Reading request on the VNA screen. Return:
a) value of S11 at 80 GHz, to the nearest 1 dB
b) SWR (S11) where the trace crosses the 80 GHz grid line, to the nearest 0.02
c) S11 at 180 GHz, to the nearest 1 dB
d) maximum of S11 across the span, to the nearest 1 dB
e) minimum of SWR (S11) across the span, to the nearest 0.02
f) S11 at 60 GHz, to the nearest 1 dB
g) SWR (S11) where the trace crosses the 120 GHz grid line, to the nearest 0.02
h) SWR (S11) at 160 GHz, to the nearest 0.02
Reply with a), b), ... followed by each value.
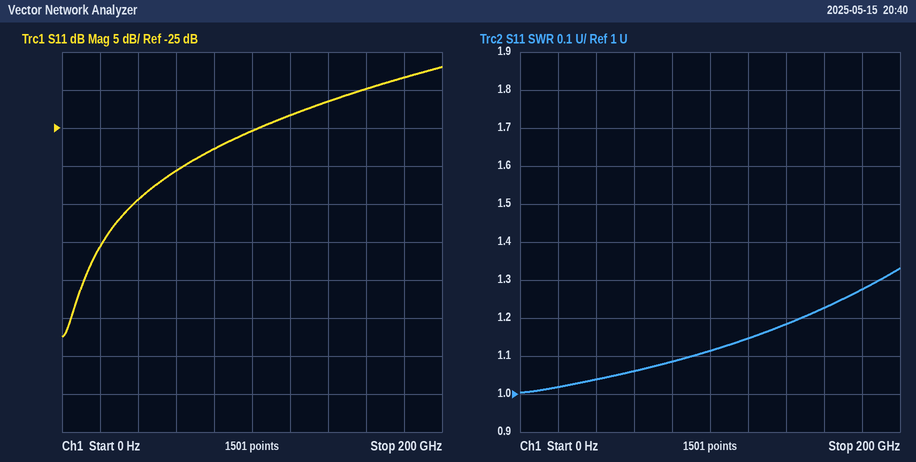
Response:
a) -28 dB
b) 1.08
c) -18 dB
d) -17 dB
e) 1.00
f) -31 dB
g) 1.14
h) 1.22
